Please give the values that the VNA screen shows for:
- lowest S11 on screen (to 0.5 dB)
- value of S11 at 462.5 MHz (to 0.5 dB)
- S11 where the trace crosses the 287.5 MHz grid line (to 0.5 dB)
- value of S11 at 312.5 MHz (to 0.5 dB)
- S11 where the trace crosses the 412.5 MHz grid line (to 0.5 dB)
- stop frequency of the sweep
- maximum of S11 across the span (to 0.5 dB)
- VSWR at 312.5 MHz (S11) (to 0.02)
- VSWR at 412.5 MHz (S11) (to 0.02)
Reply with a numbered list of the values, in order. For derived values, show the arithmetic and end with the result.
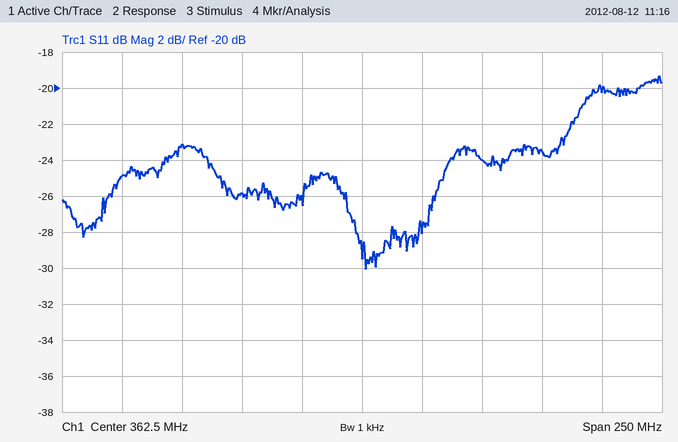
1. -30.0 dB
2. -20.0 dB
3. -23.0 dB
4. -26.0 dB
5. -24.0 dB
6. 487.5 MHz
7. -19.5 dB
8. |Γ| = 10^(-26/20) = 0.0501; VSWR = (1 + 0.0501)/(1 − 0.0501) ≈ 1.11, so 1.10 to the nearest 0.02
9. |Γ| = 10^(-24/20) = 0.0631; VSWR = (1 + 0.0631)/(1 − 0.0631) ≈ 1.13, so 1.14 to the nearest 0.02
